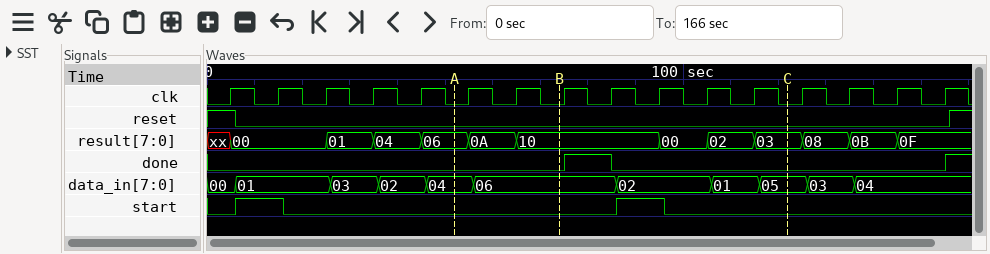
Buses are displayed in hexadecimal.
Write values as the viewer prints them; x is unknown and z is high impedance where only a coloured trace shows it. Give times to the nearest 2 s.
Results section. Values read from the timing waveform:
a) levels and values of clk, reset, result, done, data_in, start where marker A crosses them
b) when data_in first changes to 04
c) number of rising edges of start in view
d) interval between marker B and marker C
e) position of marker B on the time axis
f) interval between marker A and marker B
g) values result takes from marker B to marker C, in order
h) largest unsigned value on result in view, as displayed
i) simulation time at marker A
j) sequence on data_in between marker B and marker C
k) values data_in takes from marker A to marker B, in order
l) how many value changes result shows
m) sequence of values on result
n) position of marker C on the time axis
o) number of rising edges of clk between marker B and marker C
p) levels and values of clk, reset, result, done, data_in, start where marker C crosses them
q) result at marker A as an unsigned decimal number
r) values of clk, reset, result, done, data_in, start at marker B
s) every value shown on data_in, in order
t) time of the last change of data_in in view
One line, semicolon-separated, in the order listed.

clk=0, reset=0, result=06, done=0, data_in=04, start=0; 46 s; 2; 48 s; 74 s; 22 s; 10, 00, 02, 03; 10; 52 s; 06, 02, 01, 05; 04, 06; 12; xx, 00, 01, 04, 06, 0A, 10, 00, 02, 03, 08, 0B, 0F; 122 s; 5; clk=0, reset=0, result=03, done=0, data_in=05, start=0; 6; clk=0, reset=0, result=10, done=0, data_in=06, start=0; 00, 01, 03, 02, 04, 06, 02, 01, 05, 03, 04; 136 s
